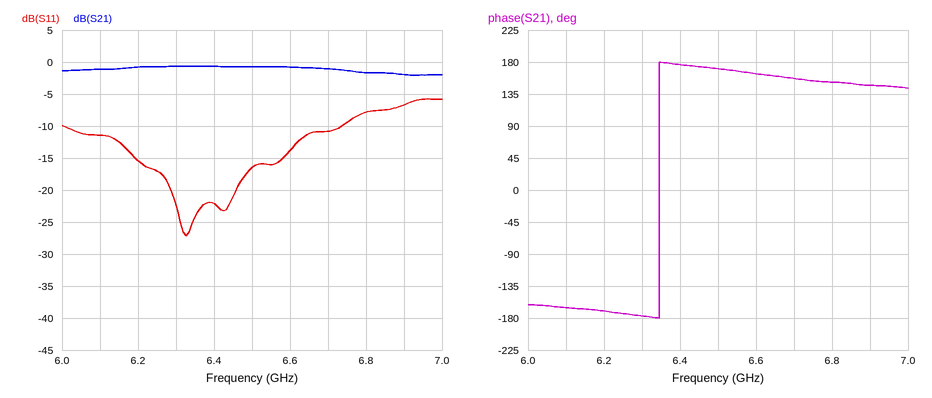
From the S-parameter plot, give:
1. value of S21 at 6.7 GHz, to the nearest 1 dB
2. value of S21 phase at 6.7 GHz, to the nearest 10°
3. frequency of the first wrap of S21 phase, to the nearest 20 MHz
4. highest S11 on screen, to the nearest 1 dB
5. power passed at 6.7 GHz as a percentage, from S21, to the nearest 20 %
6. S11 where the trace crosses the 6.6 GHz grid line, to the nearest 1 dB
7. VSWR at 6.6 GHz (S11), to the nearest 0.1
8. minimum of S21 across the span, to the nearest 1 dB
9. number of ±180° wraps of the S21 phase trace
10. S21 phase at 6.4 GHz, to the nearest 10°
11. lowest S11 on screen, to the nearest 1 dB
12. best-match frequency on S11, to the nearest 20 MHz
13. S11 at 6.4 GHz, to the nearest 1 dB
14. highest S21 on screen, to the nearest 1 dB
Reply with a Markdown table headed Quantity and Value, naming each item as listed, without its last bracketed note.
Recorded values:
| Quantity | Value |
|---|---|
| value of S21 at 6.7 GHz, to the nearest 1 dB | -1 dB |
| value of S21 phase at 6.7 GHz, to the nearest 10° | 160° |
| frequency of the first wrap of S21 phase, to the nearest 20 MHz | 6.34 GHz |
| highest S11 on screen, to the nearest 1 dB | -6 dB |
| power passed at 6.7 GHz as a percentage, from S21, to the nearest 20 % | 80 % |
| S11 where the trace crosses the 6.6 GHz grid line, to the nearest 1 dB | -14 dB |
| VSWR at 6.6 GHz (S11), to the nearest 0.1 | 1.5 |
| minimum of S21 across the span, to the nearest 1 dB | -2 dB |
| number of ±180° wraps of the S21 phase trace | 1 |
| S21 phase at 6.4 GHz, to the nearest 10° | 180° |
| lowest S11 on screen, to the nearest 1 dB | -27 dB |
| best-match frequency on S11, to the nearest 20 MHz | 6.32 GHz |
| S11 at 6.4 GHz, to the nearest 1 dB | -22 dB |
| highest S21 on screen, to the nearest 1 dB | -1 dB |
